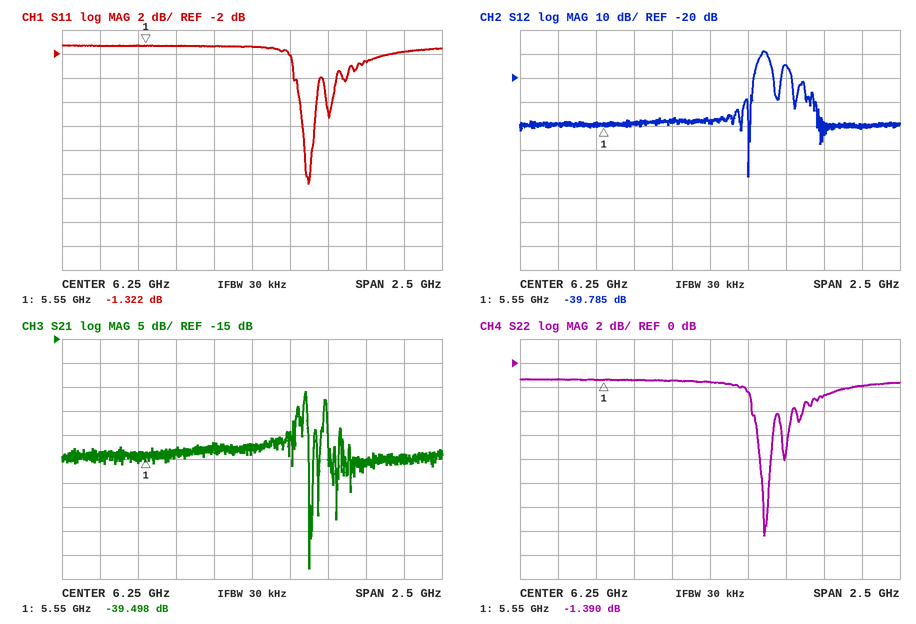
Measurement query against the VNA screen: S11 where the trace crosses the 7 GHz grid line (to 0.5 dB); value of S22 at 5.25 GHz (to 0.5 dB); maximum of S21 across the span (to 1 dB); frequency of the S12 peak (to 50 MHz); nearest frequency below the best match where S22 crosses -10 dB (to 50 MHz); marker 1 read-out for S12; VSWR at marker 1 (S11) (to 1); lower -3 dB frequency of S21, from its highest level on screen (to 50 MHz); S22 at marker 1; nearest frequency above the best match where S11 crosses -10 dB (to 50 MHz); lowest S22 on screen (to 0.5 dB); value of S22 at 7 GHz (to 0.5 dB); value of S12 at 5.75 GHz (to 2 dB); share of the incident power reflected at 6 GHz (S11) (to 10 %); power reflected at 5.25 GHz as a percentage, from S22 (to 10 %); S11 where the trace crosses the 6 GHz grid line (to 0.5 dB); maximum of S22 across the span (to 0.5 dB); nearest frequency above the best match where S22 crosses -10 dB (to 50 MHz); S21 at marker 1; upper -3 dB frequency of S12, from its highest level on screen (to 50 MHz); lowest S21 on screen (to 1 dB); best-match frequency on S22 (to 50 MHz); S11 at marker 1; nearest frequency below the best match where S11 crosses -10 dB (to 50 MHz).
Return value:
-2.5 dB
-1.5 dB
-26 dB
6.60 GHz
6.60 GHz
-39.785 dB
13
6.60 GHz
-1.390 dB
6.65 GHz
-14.5 dB
-2.5 dB
-38 dB
70 %
70 %
-1.5 dB
-1.5 dB
6.65 GHz
-39.498 dB
6.65 GHz
-63 dB
6.60 GHz
-1.322 dB
6.60 GHz
